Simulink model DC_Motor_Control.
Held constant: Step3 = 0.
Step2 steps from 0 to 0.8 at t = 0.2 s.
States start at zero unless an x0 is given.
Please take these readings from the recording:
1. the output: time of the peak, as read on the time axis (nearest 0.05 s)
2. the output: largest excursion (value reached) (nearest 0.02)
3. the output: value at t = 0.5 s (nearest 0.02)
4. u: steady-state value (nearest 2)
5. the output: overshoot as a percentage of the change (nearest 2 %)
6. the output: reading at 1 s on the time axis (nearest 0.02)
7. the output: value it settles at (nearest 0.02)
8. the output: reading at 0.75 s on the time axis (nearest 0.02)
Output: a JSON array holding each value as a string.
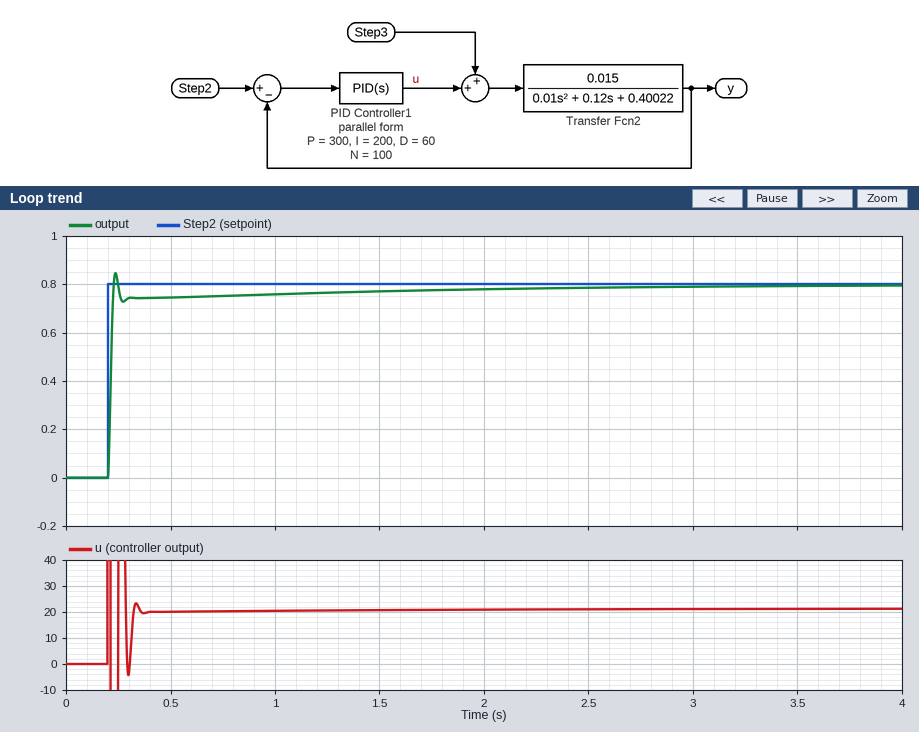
["0.25 s", "0.84", "0.74", "22", "6 %", "0.76", "0.80", "0.76"]
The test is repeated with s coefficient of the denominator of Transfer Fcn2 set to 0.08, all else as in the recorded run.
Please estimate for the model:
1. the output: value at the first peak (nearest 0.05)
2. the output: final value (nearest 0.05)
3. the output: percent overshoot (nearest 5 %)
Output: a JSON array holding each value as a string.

["0.90", "0.80", "10 %"]
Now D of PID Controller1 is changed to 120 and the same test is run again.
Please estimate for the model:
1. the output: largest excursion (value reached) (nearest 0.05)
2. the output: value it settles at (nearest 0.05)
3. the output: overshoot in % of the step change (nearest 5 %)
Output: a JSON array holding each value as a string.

["0.95", "0.80", "20 %"]
